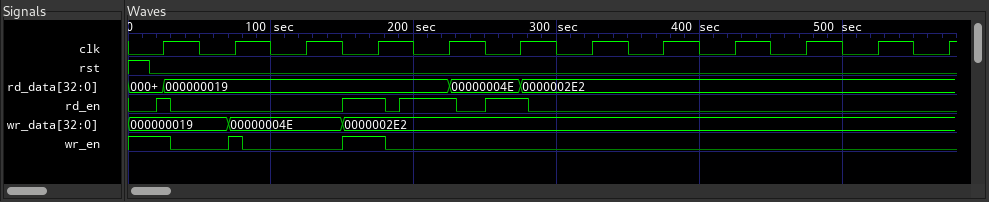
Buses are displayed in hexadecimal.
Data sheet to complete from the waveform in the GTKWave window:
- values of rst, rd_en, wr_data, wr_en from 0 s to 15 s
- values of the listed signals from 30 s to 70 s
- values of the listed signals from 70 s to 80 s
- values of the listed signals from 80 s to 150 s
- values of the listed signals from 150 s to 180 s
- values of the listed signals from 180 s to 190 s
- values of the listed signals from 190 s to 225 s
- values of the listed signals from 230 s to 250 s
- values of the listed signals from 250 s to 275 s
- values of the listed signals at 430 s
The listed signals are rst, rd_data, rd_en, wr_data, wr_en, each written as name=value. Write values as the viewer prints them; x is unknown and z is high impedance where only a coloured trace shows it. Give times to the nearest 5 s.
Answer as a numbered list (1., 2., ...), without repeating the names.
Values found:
1. rst=1, rd_en=0, wr_data=000000019, wr_en=1
2. rst=0, rd_data=000000019, rd_en=0, wr_data=000000019, wr_en=0
3. rst=0, rd_data=000000019, rd_en=0, wr_data=00000004E, wr_en=1
4. rst=0, rd_data=000000019, rd_en=0, wr_data=00000004E, wr_en=0
5. rst=0, rd_data=000000019, rd_en=1, wr_data=0000002E2, wr_en=1
6. rst=0, rd_data=000000019, rd_en=0, wr_data=0000002E2, wr_en=0
7. rst=0, rd_data=000000019, rd_en=1, wr_data=0000002E2, wr_en=0
8. rst=0, rd_data=00000004E, rd_en=0, wr_data=0000002E2, wr_en=0
9. rst=0, rd_data=00000004E, rd_en=1, wr_data=0000002E2, wr_en=0
10. rst=0, rd_data=0000002E2, rd_en=0, wr_data=0000002E2, wr_en=0
